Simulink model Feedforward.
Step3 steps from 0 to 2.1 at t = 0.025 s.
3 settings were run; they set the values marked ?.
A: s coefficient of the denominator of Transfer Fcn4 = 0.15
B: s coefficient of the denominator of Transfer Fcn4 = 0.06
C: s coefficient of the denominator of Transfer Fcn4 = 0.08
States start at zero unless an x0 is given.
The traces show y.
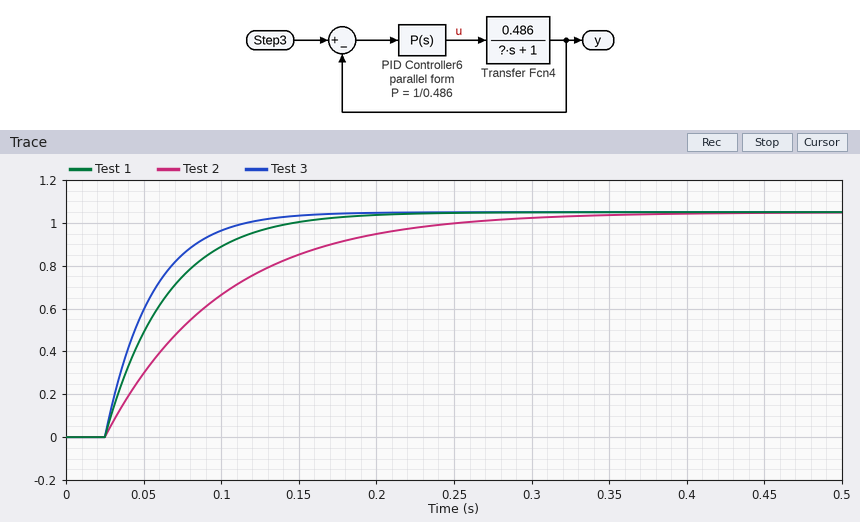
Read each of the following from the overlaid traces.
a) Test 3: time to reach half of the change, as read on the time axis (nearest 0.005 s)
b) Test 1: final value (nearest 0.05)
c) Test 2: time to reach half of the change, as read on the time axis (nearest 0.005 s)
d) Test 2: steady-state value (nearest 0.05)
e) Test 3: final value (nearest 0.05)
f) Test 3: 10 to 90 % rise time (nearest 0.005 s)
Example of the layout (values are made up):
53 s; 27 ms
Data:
0.045 s; 1.05; 0.075 s; 1.05; 1.05; 0.065 s
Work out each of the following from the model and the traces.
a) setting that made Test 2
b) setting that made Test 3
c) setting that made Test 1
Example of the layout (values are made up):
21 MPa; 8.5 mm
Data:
A; B; C
